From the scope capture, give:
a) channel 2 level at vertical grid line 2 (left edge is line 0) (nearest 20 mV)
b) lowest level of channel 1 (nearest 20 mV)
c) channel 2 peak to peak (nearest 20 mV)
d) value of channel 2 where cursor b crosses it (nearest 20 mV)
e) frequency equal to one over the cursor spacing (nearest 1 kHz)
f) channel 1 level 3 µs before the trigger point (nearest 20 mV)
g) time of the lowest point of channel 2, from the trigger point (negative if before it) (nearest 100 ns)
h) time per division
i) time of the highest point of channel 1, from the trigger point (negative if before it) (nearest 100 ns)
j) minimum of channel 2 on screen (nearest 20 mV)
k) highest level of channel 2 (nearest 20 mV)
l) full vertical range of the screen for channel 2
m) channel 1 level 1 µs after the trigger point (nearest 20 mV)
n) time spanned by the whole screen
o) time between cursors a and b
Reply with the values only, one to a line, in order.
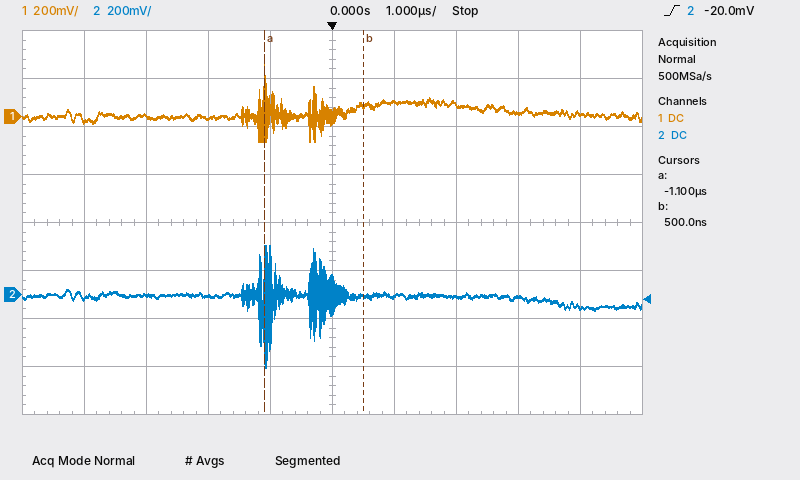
0 mV
-100 mV
500 mV
0 mV
625 kHz
0 mV
-1.1 µs
1 µs
-1.1 µs
-300 mV
200 mV
1.6 V
60 mV
10 µs
1.6 µs
